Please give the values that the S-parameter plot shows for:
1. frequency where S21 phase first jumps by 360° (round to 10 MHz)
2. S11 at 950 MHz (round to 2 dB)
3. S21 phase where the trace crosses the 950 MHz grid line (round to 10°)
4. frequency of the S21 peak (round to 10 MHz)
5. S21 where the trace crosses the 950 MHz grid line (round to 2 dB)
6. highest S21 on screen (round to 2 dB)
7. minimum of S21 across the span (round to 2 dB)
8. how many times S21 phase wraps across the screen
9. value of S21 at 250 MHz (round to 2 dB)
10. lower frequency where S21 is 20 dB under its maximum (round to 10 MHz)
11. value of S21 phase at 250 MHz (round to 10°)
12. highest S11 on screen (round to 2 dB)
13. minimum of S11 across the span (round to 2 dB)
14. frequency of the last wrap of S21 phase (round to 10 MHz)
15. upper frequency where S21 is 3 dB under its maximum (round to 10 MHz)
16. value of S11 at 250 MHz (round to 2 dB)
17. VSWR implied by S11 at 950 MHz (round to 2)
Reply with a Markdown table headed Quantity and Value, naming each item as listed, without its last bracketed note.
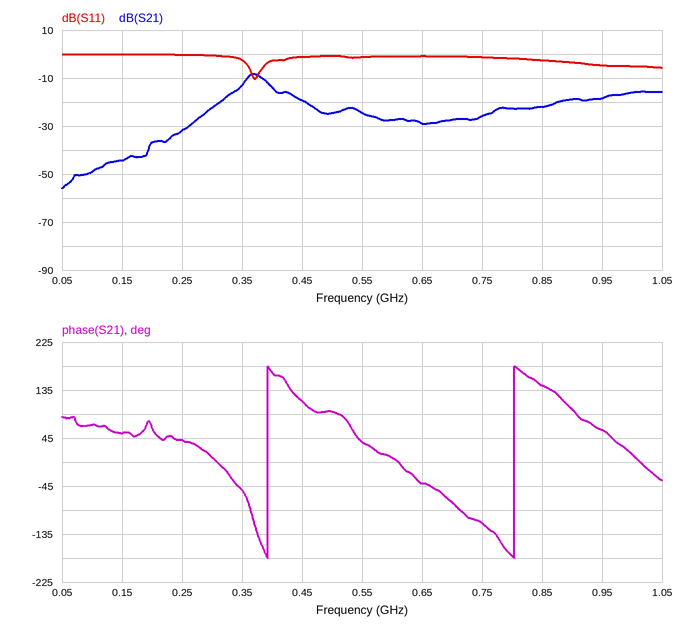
| Quantity | Value |
|---|---|
| frequency where S21 phase first jumps by 360° | 390 MHz |
| S11 at 950 MHz | -4 dB |
| S21 phase where the trace crosses the 950 MHz grid line | 60° |
| frequency of the S21 peak | 370 MHz |
| S21 where the trace crosses the 950 MHz grid line | -18 dB |
| highest S21 on screen | -8 dB |
| minimum of S21 across the span | -56 dB |
| how many times S21 phase wraps across the screen | 2 |
| value of S21 at 250 MHz | -32 dB |
| lower frequency where S21 is 20 dB under its maximum | 270 MHz |
| value of S21 phase at 250 MHz | 40° |
| highest S11 on screen | 0 dB |
| minimum of S11 across the span | -10 dB |
| frequency of the last wrap of S21 phase | 800 MHz |
| upper frequency where S21 is 3 dB under its maximum | 390 MHz |
| value of S11 at 250 MHz | 0 dB |
| VSWR implied by S11 at 950 MHz | 4 |
